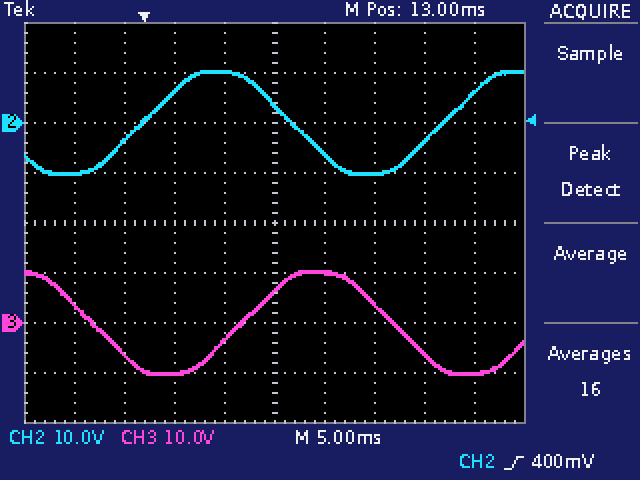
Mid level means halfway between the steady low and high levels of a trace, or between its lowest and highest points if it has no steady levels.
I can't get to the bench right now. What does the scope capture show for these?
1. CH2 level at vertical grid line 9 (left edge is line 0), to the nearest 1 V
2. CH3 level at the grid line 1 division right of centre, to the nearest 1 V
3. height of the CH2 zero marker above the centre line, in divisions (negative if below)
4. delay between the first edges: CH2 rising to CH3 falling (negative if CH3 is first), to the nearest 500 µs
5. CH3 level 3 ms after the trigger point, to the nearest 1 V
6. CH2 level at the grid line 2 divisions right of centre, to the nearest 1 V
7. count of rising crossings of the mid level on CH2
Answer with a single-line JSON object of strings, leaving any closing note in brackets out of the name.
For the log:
{"CH2 level at vertical grid line 9 (left edge is line 0), to the nearest 1 V": "6 V", "CH3 level at the grid line 1 division right of centre, to the nearest 1 V": "10 V", "height of the CH2 zero marker above the centre line, in divisions": "+2.0 div", "delay between the first edges: CH2 rising to CH3 falling (negative if CH3 is first), to the nearest 500 µs": "-5.0 ms", "CH3 level 3 ms after the trigger point, to the nearest 1 V": "-10 V", "CH2 level at the grid line 2 divisions right of centre, to the nearest 1 V": "-10 V", "count of rising crossings of the mid level on CH2": "2"}
